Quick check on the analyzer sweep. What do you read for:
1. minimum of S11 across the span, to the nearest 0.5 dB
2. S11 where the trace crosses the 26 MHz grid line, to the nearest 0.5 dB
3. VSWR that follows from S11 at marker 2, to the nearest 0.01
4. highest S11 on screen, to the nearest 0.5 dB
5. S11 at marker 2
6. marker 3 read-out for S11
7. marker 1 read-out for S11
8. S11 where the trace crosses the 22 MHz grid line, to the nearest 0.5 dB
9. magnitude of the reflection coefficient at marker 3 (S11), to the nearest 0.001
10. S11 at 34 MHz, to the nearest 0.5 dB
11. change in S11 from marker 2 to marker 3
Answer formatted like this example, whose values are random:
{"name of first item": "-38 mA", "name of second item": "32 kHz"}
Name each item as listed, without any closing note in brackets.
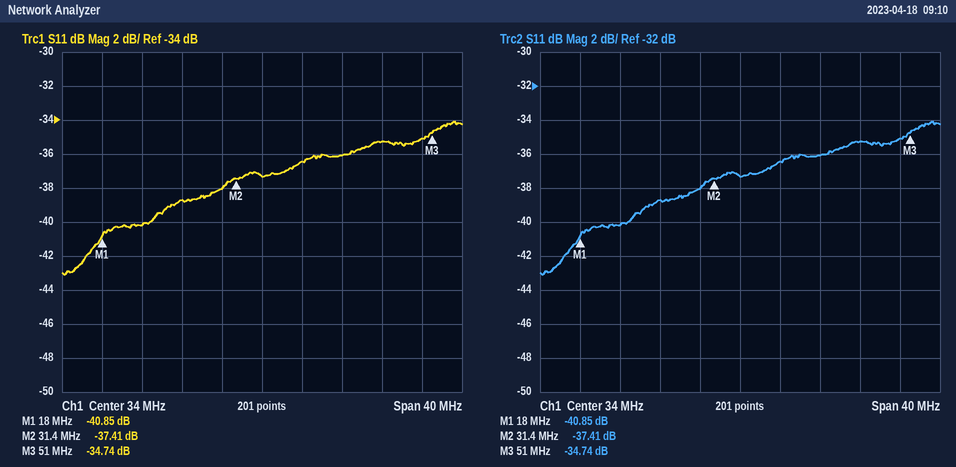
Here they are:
{"minimum of S11 across the span, to the nearest 0.5 dB": "-43.0 dB", "S11 where the trace crosses the 26 MHz grid line, to the nearest 0.5 dB": "-38.5 dB", "VSWR that follows from S11 at marker 2, to the nearest 0.01": "1.03", "highest S11 on screen, to the nearest 0.5 dB": "-34.0 dB", "S11 at marker 2": "-37.41 dB", "marker 3 read-out for S11": "-34.74 dB", "marker 1 read-out for S11": "-40.85 dB", "S11 where the trace crosses the 22 MHz grid line, to the nearest 0.5 dB": "-40.0 dB", "magnitude of the reflection coefficient at marker 3 (S11), to the nearest 0.001": "0.018", "S11 at 34 MHz, to the nearest 0.5 dB": "-37.5 dB", "change in S11 from marker 2 to marker 3": "2.67 dB"}
